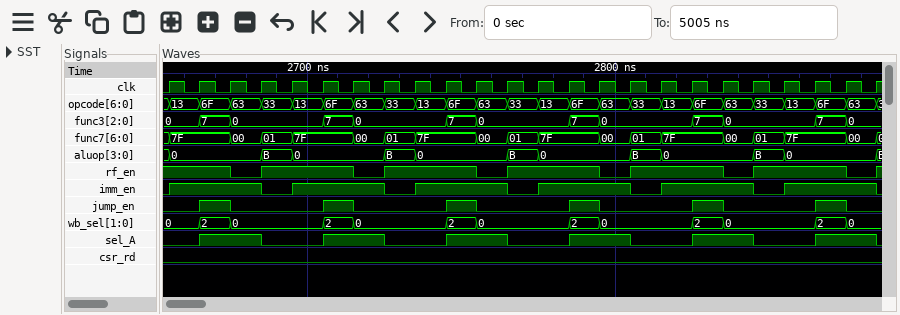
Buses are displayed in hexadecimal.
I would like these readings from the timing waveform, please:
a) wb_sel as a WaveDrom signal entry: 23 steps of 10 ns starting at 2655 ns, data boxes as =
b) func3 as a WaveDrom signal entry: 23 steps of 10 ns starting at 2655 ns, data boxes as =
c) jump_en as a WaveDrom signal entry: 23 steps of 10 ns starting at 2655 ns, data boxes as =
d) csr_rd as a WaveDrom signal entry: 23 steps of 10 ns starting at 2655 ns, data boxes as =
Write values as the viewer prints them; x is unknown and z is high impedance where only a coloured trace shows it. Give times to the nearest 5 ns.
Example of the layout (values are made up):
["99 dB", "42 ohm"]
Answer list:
["{name: 'wb_sel', wave: '===..==..==..==..==..==', data: '0 2 0 2 0 2 0 2 0 2 0 2 0'}", "{name: 'func3', wave: '===..==..==..==..==..==', data: '0 7 0 7 0 7 0 7 0 7 0 7 0'}", "{name: 'jump_en', wave: '010..10..10..10..10..10'}", "{name: 'csr_rd', wave: '0......................'}"]
